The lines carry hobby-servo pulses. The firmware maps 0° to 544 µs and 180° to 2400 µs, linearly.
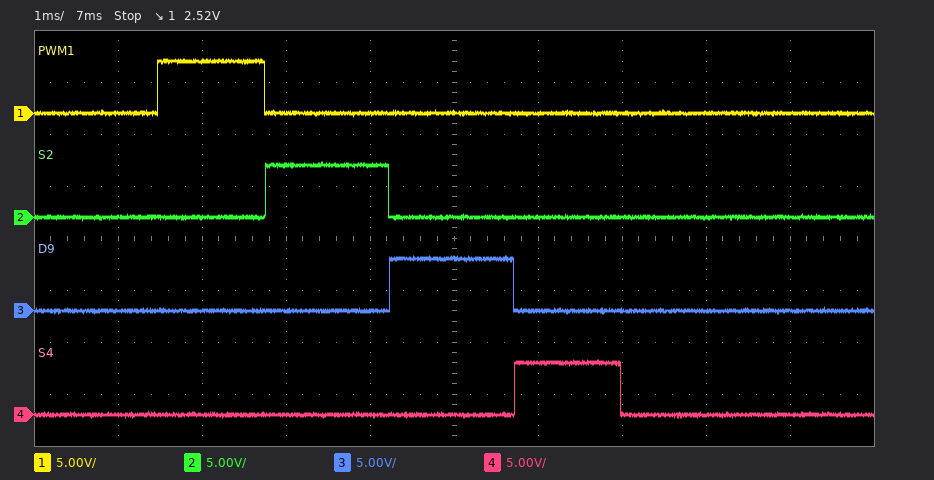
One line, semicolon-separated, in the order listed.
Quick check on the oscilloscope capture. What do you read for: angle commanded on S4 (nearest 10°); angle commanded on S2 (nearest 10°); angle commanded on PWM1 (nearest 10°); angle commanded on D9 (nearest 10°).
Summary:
70°; 90°; 70°; 90°
